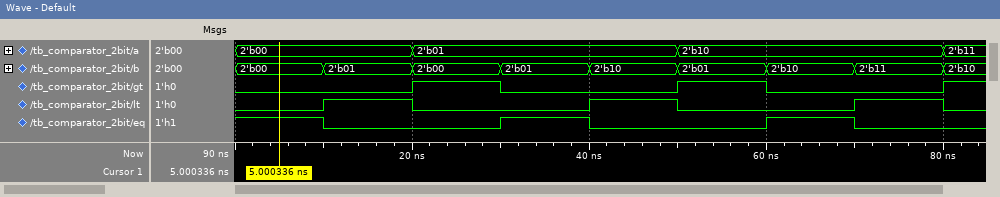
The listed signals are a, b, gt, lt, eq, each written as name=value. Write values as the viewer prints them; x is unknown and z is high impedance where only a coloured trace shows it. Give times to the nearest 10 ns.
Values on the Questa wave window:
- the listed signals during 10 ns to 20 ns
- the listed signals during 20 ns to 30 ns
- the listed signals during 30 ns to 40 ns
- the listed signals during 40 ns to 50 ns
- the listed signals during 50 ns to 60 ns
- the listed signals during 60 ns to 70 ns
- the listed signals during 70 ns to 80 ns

a=2'b00, b=2'b01, gt=0, lt=1, eq=0
a=2'b01, b=2'b00, gt=1, lt=0, eq=0
a=2'b01, b=2'b01, gt=0, lt=0, eq=1
a=2'b01, b=2'b10, gt=0, lt=1, eq=0
a=2'b10, b=2'b01, gt=1, lt=0, eq=0
a=2'b10, b=2'b10, gt=0, lt=0, eq=1
a=2'b10, b=2'b11, gt=0, lt=1, eq=0
